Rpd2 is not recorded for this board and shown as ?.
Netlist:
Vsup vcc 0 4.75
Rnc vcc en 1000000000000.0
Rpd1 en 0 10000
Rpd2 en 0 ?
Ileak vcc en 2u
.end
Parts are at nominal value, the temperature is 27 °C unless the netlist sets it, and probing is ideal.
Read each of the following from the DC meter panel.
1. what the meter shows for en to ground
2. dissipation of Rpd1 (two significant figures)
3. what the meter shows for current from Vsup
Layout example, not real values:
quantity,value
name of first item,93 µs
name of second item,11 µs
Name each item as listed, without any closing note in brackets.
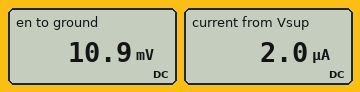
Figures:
quantity,value
what the meter shows for en to ground,10.9 mV
dissipation of Rpd1,12 nW
what the meter shows for current from Vsup,2.0 µA
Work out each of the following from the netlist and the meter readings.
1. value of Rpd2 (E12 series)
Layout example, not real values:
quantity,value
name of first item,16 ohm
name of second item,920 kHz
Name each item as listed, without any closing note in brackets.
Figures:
quantity,value
value of Rpd2,12 kΩ
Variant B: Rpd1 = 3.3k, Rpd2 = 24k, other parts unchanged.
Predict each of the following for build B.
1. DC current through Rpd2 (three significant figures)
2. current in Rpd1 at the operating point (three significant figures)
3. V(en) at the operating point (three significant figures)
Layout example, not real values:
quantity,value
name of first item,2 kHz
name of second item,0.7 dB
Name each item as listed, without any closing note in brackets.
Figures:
quantity,value
DC current through Rpd2,242 nA
current in Rpd1 at the operating point,1.76 µA
V(en) at the operating point,5.80 mV
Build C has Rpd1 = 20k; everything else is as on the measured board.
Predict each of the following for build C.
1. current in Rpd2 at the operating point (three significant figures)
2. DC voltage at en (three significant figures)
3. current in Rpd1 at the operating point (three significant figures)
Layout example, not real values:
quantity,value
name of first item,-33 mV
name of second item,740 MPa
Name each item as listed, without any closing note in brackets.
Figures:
quantity,value
current in Rpd2 at the operating point,1.25 µA
DC voltage at en,15.0 mV
current in Rpd1 at the operating point,750 nA
